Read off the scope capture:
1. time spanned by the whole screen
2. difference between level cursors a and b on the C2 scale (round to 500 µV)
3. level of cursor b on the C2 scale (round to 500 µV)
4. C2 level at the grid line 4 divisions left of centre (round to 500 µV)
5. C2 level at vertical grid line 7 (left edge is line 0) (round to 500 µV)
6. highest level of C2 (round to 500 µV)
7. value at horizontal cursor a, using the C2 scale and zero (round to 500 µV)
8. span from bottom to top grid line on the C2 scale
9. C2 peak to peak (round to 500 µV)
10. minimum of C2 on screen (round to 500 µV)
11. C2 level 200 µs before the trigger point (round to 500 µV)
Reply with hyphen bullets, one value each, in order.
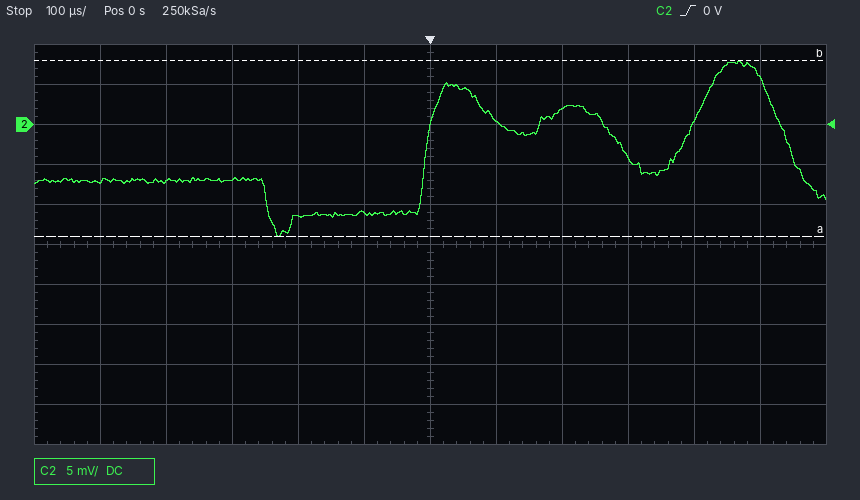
- 1.2 ms
- 22.0 mV
- 8.0 mV
- -7.0 mV
- 500 µV
- 8.0 mV
- -14.0 mV
- 50 mV
- 22.0 mV
- -14.0 mV
- -11.5 mV
